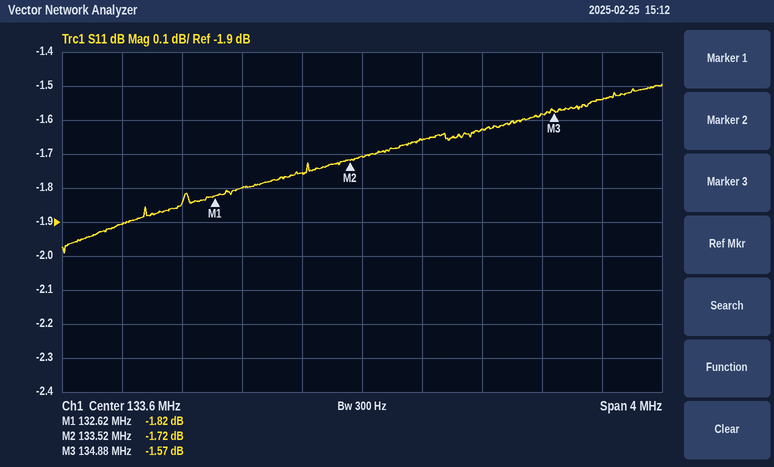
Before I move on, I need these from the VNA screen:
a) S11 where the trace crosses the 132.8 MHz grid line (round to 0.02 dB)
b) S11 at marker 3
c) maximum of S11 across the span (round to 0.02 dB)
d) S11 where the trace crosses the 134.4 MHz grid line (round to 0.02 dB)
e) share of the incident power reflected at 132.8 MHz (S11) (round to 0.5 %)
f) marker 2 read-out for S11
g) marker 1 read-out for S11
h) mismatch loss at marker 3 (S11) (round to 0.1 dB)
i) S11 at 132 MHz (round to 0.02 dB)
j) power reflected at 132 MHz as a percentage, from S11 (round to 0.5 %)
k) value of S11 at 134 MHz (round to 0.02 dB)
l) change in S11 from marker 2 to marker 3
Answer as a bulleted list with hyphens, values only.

- -1.80 dB
- -1.57 dB
- -1.50 dB
- -1.62 dB
- 66.0 %
- -1.72 dB
- -1.82 dB
- 5.2 dB
- -1.90 dB
- 64.5 %
- -1.66 dB
- 0.15 dB
